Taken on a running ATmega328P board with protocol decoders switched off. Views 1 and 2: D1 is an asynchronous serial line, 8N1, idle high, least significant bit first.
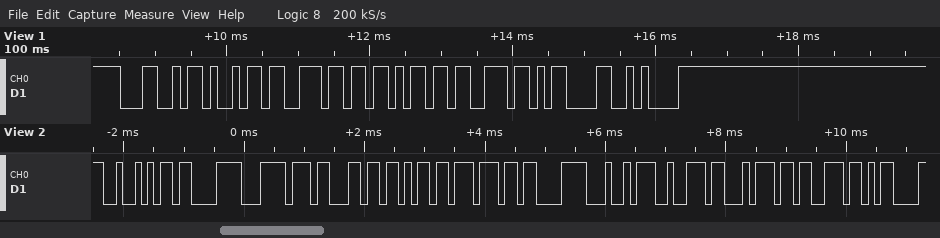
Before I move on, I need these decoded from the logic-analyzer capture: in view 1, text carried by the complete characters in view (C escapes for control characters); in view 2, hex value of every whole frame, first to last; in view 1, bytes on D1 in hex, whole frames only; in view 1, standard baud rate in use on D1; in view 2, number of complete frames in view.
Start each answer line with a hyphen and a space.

- "Links\r\n"
- 52 C3 BC 63 6B 77 C3 A4 72 74 73 0D
- 4C 69 6E 6B 73 0D 0A
- 9600 baud
- 12
